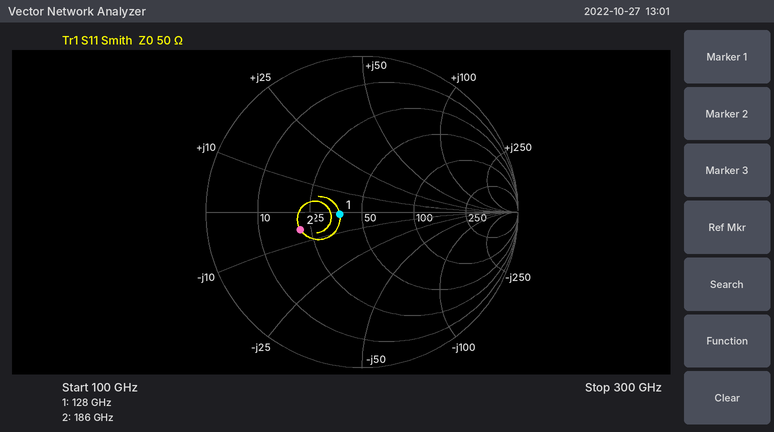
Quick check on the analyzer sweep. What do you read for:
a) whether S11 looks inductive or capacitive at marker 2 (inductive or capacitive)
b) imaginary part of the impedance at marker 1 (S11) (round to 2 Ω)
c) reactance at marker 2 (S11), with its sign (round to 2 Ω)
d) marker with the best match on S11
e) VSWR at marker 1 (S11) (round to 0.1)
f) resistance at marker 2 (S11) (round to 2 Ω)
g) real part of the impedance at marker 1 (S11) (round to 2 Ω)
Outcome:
capacitive
-2 Ω
-6 Ω
marker 1
1.3
22 Ω
38 Ω
